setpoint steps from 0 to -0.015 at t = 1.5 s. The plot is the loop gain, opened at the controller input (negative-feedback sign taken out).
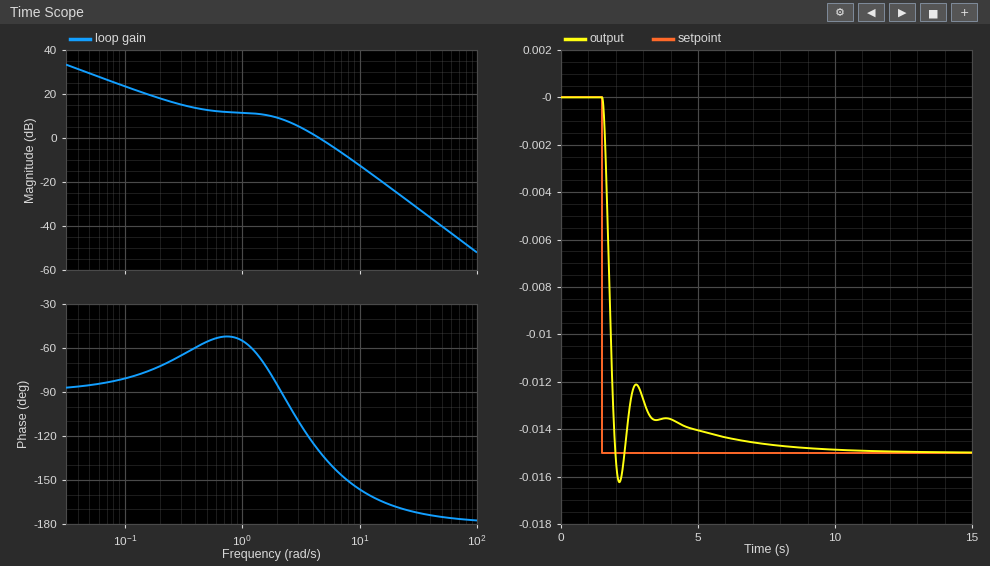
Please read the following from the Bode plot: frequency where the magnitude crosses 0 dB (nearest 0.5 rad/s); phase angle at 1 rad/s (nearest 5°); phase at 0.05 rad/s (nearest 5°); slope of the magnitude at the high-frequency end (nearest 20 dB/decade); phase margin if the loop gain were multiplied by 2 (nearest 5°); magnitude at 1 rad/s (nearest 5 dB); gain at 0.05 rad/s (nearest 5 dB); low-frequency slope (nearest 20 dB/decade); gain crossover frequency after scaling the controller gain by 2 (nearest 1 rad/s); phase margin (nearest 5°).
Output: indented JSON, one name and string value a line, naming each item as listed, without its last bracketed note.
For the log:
{
  "frequency where the magnitude crosses 0 dB": "4.5 rad/s",
  "phase angle at 1 rad/s": "-55°",
  "phase at 0.05 rad/s": "-85°",
  "slope of the magnitude at the high-frequency end": "-40 dB/decade",
  "phase margin if the loop gain were multiplied by 2": "35°",
  "magnitude at 1 rad/s": "10 dB",
  "gain at 0.05 rad/s": "30 dB",
  "low-frequency slope": "-20 dB/decade",
  "gain crossover frequency after scaling the controller gain by 2": "7 rad/s",
  "phase margin": "50°"
}
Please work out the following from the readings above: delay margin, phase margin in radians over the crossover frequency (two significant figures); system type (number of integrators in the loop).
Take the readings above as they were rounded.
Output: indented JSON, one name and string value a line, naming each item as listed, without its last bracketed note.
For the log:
{
  "delay margin, phase margin in radians over the crossover frequency": "0.19 s",
  "system type": "1"
}
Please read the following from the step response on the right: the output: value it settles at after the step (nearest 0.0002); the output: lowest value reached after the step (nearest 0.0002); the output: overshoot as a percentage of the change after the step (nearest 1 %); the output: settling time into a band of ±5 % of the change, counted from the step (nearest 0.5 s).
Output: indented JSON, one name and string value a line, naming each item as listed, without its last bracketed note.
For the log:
{
  "the output: value it settles at after the step": "-0.0150",
  "the output: lowest value reached after the step": "-0.0162",
  "the output: overshoot as a percentage of the change after the step": "8 %",
  "the output: settling time into a band of ±5 % of the change, counted from the step": "4.0 s"
}
